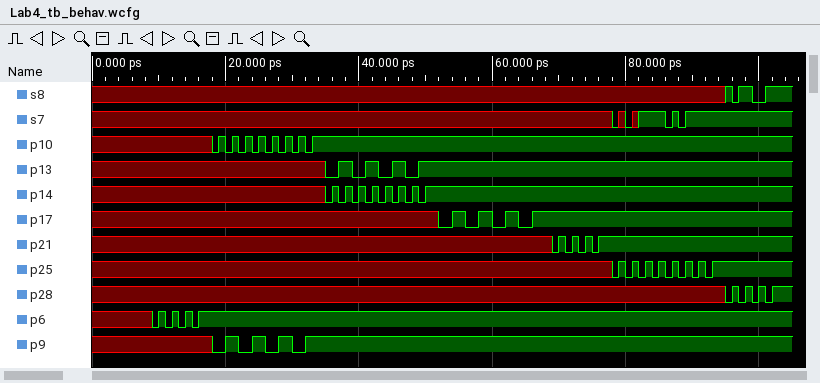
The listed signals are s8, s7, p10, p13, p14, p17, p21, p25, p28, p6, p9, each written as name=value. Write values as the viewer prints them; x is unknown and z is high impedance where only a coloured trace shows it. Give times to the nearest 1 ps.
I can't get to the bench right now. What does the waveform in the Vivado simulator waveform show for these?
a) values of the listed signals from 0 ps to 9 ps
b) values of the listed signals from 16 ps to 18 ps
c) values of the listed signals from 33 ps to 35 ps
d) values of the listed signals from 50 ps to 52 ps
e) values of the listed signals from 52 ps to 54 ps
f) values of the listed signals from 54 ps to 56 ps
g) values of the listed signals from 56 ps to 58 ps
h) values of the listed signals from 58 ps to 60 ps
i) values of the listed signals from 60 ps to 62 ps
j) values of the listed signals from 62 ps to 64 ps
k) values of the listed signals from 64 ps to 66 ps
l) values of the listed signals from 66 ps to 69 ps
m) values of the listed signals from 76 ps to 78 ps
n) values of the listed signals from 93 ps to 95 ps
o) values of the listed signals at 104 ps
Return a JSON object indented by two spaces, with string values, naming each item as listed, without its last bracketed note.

{
  "values of the listed signals from 0 ps to 9 ps": "s8=x, s7=x, p10=x, p13=x, p14=x, p17=x, p21=x, p25=x, p28=x, p6=x, p9=x",
  "values of the listed signals from 16 ps to 18 ps": "s8=x, s7=x, p10=x, p13=x, p14=x, p17=x, p21=x, p25=x, p28=x, p6=1, p9=x",
  "values of the listed signals from 33 ps to 35 ps": "s8=x, s7=x, p10=1, p13=x, p14=x, p17=x, p21=x, p25=x, p28=x, p6=1, p9=1",
  "values of the listed signals from 50 ps to 52 ps": "s8=x, s7=x, p10=1, p13=1, p14=1, p17=x, p21=x, p25=x, p28=x, p6=1, p9=1",
  "values of the listed signals from 52 ps to 54 ps": "s8=x, s7=x, p10=1, p13=1, p14=1, p17=0, p21=x, p25=x, p28=x, p6=1, p9=1",
  "values of the listed signals from 54 ps to 56 ps": "s8=x, s7=x, p10=1, p13=1, p14=1, p17=1, p21=x, p25=x, p28=x, p6=1, p9=1",
  "values of the listed signals from 56 ps to 58 ps": "s8=x, s7=x, p10=1, p13=1, p14=1, p17=0, p21=x, p25=x, p28=x, p6=1, p9=1",
  "values of the listed signals from 58 ps to 60 ps": "s8=x, s7=x, p10=1, p13=1, p14=1, p17=1, p21=x, p25=x, p28=x, p6=1, p9=1",
  "values of the listed signals from 60 ps to 62 ps": "s8=x, s7=x, p10=1, p13=1, p14=1, p17=0, p21=x, p25=x, p28=x, p6=1, p9=1",
  "values of the listed signals from 62 ps to 64 ps": "s8=x, s7=x, p10=1, p13=1, p14=1, p17=1, p21=x, p25=x, p28=x, p6=1, p9=1",
  "values of the listed signals from 64 ps to 66 ps": "s8=x, s7=x, p10=1, p13=1, p14=1, p17=0, p21=x, p25=x, p28=x, p6=1, p9=1",
  "values of the listed signals from 66 ps to 69 ps": "s8=x, s7=x, p10=1, p13=1, p14=1, p17=1, p21=x, p25=x, p28=x, p6=1, p9=1",
  "values of the listed signals from 76 ps to 78 ps": "s8=x, s7=x, p10=1, p13=1, p14=1, p17=1, p21=1, p25=x, p28=x, p6=1, p9=1",
  "values of the listed signals from 93 ps to 95 ps": "s8=x, s7=1, p10=1, p13=1, p14=1, p17=1, p21=1, p25=1, p28=x, p6=1, p9=1",
  "values of the listed signals at 104 ps": "s8=1, s7=1, p10=1, p13=1, p14=1, p17=1, p21=1, p25=1, p28=1, p6=1, p9=1"
}
